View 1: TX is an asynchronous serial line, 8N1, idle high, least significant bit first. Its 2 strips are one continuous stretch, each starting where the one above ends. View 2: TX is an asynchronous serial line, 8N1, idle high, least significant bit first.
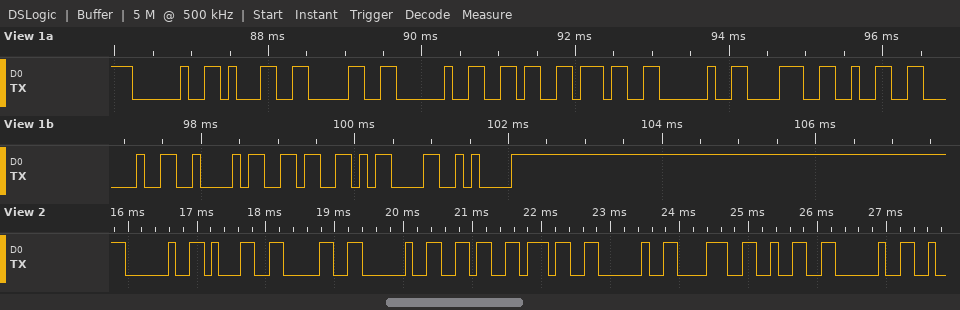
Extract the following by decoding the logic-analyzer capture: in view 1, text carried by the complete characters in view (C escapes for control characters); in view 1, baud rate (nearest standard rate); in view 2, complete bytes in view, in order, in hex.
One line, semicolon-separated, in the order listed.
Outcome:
" 10 67 82 B6\r\n"; 9600 baud; 20 31 30 20 36 37 20 38 32 20
